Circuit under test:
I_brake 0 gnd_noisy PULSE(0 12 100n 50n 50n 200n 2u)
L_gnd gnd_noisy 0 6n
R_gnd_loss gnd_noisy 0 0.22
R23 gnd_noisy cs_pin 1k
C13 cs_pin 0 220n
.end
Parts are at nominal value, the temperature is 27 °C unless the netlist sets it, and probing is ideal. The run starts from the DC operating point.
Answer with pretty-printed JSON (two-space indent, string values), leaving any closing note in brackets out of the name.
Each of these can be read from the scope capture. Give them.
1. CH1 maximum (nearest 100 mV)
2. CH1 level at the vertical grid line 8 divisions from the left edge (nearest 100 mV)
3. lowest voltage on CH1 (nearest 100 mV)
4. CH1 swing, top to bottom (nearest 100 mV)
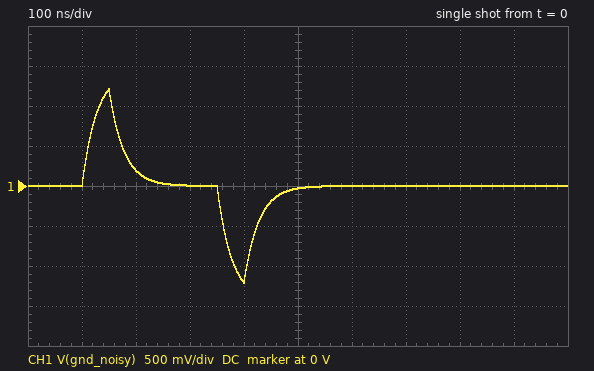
{
  "CH1 maximum": "1.2 V",
  "CH1 level at the vertical grid line 8 divisions from the left edge": "0 V",
  "lowest voltage on CH1": "-1.2 V",
  "CH1 swing, top to bottom": "2.4 V"
}
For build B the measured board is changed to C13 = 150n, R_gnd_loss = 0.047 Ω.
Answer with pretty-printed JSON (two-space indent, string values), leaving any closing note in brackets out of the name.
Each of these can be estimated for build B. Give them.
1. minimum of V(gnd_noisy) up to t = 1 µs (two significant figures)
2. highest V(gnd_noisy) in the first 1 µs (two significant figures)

{
  "minimum of V(gnd_noisy) up to t = 1 µs": "-400 mV",
  "highest V(gnd_noisy) in the first 1 µs": "470 mV"
}
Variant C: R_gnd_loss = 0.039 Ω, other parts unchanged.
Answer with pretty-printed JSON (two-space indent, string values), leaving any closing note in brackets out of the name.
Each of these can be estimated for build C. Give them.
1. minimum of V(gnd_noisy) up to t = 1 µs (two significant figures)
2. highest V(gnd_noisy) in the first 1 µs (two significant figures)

{
  "minimum of V(gnd_noisy) up to t = 1 µs": "-320 mV",
  "highest V(gnd_noisy) in the first 1 µs": "400 mV"
}
